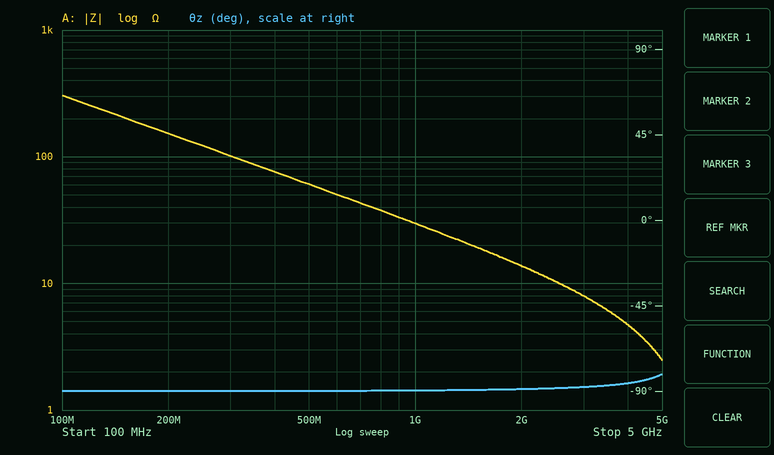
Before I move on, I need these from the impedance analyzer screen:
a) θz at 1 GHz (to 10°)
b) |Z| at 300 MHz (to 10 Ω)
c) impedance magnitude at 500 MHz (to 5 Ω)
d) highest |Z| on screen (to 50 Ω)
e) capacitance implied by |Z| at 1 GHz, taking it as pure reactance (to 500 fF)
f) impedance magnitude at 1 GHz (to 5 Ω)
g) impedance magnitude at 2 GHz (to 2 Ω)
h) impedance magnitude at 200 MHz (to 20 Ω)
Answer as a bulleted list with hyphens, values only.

- -90°
- 100 Ω
- 60 Ω
- 300 Ω
- 5.5 pF
- 30 Ω
- 14 Ω
- 160 Ω
